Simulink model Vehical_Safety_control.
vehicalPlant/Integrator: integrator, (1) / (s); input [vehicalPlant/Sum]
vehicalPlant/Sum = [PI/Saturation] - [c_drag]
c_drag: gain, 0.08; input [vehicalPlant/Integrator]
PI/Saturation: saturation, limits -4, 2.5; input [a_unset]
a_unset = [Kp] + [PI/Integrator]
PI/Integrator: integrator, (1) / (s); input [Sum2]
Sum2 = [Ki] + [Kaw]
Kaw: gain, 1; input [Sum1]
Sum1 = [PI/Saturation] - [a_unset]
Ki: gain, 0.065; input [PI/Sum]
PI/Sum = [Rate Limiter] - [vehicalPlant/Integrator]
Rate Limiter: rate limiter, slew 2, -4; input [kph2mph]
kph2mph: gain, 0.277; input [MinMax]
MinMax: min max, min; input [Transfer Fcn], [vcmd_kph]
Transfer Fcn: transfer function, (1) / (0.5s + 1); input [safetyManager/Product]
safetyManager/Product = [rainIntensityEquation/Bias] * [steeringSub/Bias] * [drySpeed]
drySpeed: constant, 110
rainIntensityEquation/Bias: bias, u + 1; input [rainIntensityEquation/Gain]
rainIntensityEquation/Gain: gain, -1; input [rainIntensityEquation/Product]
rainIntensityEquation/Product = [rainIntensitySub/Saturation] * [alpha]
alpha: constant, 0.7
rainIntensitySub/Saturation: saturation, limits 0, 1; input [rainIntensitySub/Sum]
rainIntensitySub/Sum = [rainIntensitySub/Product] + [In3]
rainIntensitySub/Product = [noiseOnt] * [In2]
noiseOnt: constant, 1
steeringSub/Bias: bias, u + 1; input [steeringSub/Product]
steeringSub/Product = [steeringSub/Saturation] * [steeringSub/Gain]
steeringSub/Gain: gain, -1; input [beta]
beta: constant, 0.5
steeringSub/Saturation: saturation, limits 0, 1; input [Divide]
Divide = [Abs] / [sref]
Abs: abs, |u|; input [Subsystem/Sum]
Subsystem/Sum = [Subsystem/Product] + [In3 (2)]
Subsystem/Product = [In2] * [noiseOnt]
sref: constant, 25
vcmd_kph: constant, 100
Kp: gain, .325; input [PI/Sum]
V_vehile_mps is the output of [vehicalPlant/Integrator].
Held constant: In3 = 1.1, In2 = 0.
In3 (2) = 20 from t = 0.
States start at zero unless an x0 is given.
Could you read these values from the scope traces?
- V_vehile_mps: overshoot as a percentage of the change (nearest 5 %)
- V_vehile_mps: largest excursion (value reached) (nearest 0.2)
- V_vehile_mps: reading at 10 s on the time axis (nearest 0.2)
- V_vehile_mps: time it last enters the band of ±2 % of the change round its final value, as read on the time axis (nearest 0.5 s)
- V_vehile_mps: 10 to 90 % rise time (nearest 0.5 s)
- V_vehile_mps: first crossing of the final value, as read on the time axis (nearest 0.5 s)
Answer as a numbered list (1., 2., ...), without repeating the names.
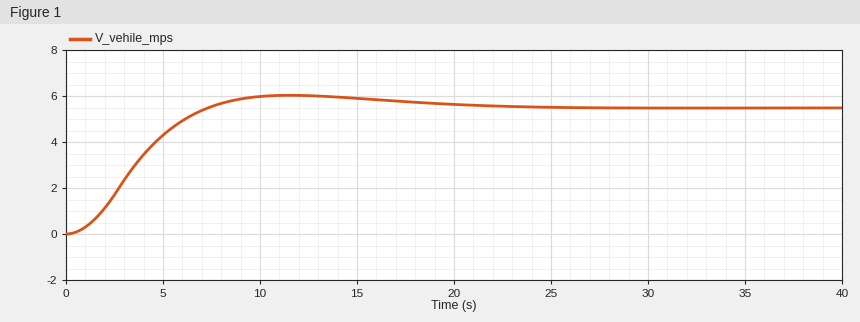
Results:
1. 10 %
2. 6.0
3. 6.0
4. 21.0 s
5. 4.5 s
6. 7.5 s
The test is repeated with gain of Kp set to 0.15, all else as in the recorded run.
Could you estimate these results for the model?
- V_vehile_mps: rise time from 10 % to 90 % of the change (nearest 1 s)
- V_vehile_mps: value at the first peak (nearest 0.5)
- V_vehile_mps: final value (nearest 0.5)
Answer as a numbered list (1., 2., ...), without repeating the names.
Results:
1. 5 s
2. 7.0
3. 5.5
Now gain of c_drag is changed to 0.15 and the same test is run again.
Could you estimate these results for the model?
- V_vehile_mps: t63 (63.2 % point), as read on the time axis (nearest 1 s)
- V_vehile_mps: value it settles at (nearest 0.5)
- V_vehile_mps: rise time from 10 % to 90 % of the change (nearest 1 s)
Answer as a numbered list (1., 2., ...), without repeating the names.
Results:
1. 4 s
2. 5.5
3. 6 s
